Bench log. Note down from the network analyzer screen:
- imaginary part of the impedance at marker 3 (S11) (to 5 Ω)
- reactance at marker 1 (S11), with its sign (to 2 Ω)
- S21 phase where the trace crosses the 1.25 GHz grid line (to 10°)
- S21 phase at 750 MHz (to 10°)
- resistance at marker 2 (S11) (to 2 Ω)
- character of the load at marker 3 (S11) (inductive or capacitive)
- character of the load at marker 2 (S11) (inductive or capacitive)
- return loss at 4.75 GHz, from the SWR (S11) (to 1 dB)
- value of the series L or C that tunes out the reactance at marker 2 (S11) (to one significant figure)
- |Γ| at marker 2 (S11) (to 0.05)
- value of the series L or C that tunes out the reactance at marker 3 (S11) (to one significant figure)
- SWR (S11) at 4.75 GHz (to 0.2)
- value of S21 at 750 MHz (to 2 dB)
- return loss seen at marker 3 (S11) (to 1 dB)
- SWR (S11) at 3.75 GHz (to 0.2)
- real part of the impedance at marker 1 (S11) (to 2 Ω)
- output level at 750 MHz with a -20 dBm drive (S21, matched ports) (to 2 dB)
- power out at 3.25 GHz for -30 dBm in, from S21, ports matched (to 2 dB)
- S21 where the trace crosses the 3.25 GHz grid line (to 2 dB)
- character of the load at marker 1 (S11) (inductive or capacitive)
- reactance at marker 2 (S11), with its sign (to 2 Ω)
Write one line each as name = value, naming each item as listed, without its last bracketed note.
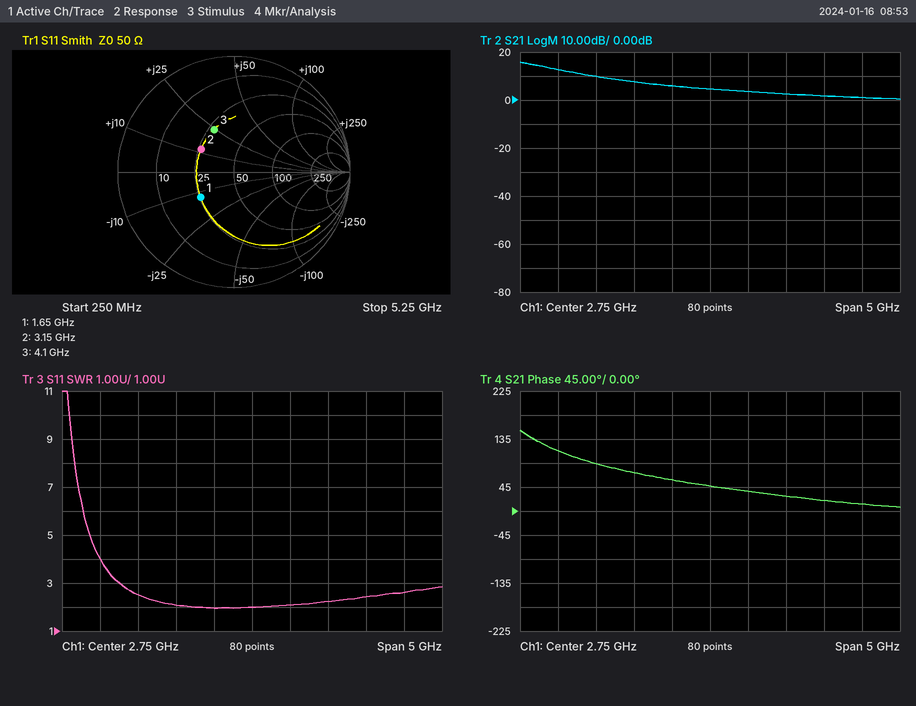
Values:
imaginary part of the impedance at marker 3 (S11) = +25 Ω
reactance at marker 1 (S11), with its sign = -12 Ω
S21 phase where the trace crosses the 1.25 GHz grid line = 90°
S21 phase at 750 MHz = 110°
resistance at marker 2 (S11) = 26 Ω
character of the load at marker 3 (S11) = inductive
character of the load at marker 2 (S11) = inductive
return loss at 4.75 GHz, from the SWR (S11) = 7 dB
value of the series L or C that tunes out the reactance at marker 2 (S11) = 4 pF
|Γ| at marker 2 (S11) = 0.35
value of the series L or C that tunes out the reactance at marker 3 (S11) = 2 pF
SWR (S11) at 4.75 GHz = 2.6
value of S21 at 750 MHz = 12 dB
return loss seen at marker 3 (S11) = 8 dB
SWR (S11) at 3.75 GHz = 2.2
real part of the impedance at marker 1 (S11) = 26 Ω
output level at 750 MHz with a -20 dBm drive (S21, matched ports) = -8 dBm
power out at 3.25 GHz for -30 dBm in, from S21, ports matched = -26 dBm
S21 where the trace crosses the 3.25 GHz grid line = 4 dB
character of the load at marker 1 (S11) = capacitive
reactance at marker 2 (S11), with its sign = +12 Ω
